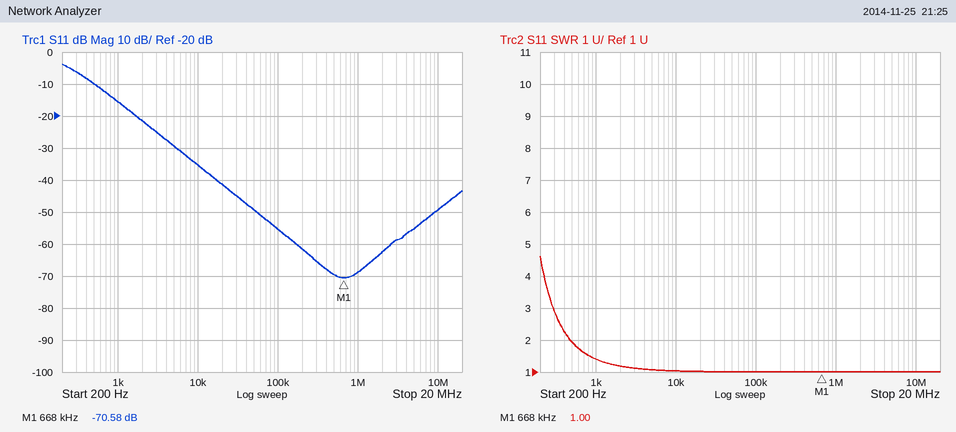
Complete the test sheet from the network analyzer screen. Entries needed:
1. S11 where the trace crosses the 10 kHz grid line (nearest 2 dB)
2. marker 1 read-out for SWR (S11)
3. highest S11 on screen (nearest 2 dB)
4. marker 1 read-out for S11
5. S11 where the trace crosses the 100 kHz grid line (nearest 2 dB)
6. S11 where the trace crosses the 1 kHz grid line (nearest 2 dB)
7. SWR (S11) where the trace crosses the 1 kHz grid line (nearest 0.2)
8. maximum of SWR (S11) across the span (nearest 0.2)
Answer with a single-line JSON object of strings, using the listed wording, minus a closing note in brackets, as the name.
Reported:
{"S11 where the trace crosses the 10 kHz grid line": "-36 dB", "marker 1 read-out for SWR": "1.00", "highest S11 on screen": "-4 dB", "marker 1 read-out for S11": "-70.58 dB", "S11 where the trace crosses the 100 kHz grid line": "-56 dB", "S11 where the trace crosses the 1 kHz grid line": "-16 dB", "SWR (S11) where the trace crosses the 1 kHz grid line": "1.4", "maximum of SWR (S11) across the span": "4.6"}
